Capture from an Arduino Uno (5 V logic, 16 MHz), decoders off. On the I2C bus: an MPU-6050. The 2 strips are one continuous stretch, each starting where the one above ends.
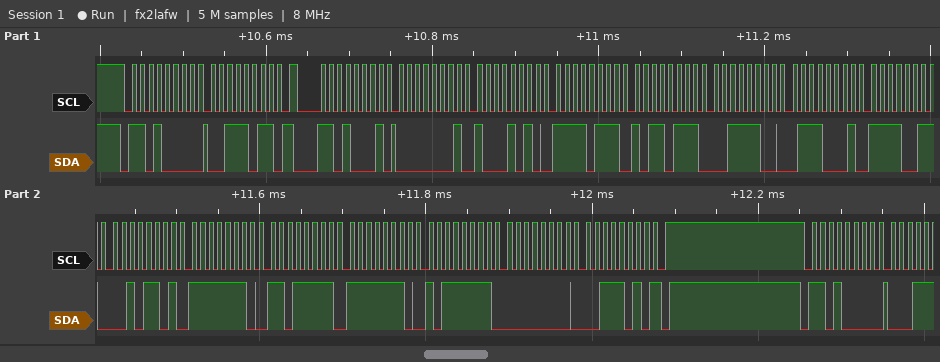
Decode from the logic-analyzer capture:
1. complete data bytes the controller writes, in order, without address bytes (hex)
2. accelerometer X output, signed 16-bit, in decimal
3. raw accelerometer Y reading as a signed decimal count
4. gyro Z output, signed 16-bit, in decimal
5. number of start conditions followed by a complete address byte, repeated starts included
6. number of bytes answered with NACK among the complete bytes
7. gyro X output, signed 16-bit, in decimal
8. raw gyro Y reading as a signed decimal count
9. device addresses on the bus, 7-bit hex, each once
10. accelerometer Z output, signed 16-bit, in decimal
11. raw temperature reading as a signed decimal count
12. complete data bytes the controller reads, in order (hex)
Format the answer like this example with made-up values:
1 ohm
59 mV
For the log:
3B
394
-2121
58
3
1
-289
-321
0x68
15473
-3283
01 8A F7 B7 3C 71 F3 2D FE DF FE BF 00 3A
